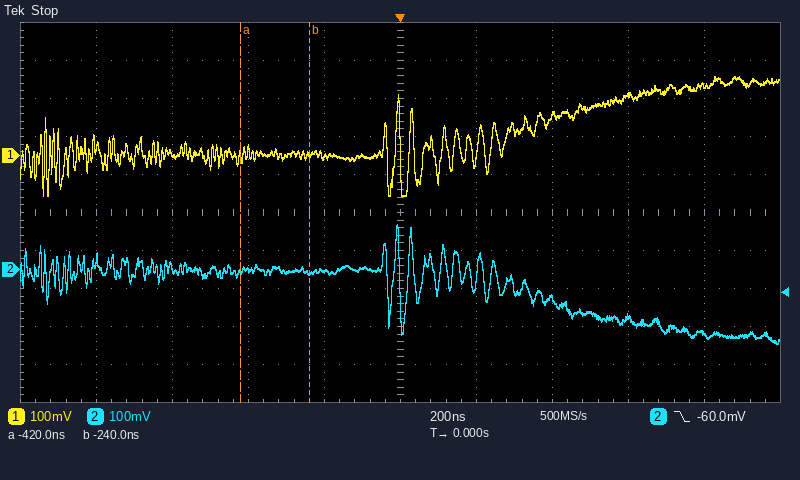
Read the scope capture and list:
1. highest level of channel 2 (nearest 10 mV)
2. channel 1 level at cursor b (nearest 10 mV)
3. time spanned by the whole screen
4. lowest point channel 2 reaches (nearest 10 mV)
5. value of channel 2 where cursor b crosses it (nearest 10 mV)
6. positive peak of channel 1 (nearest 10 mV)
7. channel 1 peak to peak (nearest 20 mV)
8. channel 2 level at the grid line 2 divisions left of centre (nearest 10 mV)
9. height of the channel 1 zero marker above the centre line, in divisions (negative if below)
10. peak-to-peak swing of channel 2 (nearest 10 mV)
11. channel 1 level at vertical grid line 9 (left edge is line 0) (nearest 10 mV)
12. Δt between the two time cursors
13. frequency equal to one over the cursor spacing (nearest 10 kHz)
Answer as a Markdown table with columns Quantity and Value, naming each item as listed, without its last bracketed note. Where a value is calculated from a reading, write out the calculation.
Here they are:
| Quantity | Value |
|---|---|
| highest level of channel 2 | 120 mV |
| channel 1 level at cursor b | 0 mV |
| time spanned by the whole screen | 2 µs |
| lowest point channel 2 reaches | -190 mV |
| value of channel 2 where cursor b crosses it | -10 mV |
| positive peak of channel 1 | 210 mV |
| channel 1 peak to peak | 320 mV |
| channel 2 level at the grid line 2 divisions left of centre | 0 mV |
| height of the channel 1 zero marker above the centre line, in divisions | +1.5 div |
| peak-to-peak swing of channel 2 | 120 mV − (-190 mV) = 310 mV |
| channel 1 level at vertical grid line 9 (left edge is line 0) | 180 mV |
| Δt between the two time cursors | -240 ns − (-420 ns) = 180 ns |
| frequency equal to one over the cursor spacing | 1 / 180 ns ≈ 5.56 MHz |
